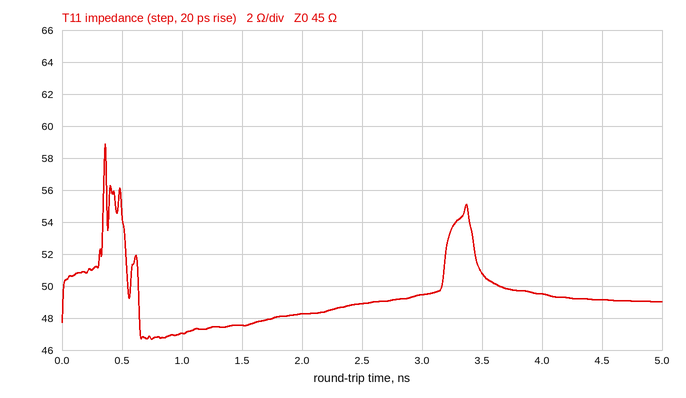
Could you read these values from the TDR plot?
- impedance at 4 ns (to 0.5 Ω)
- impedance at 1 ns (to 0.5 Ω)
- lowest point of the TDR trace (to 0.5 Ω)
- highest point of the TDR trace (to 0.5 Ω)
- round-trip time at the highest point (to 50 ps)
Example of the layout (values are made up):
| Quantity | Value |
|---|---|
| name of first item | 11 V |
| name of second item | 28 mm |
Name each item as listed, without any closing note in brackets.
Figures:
| Quantity | Value |
|---|---|
| impedance at 4 ns | 49.5 Ω |
| impedance at 1 ns | 47.0 Ω |
| lowest point of the TDR trace | 46.5 Ω |
| highest point of the TDR trace | 59.0 Ω |
| round-trip time at the highest point | 350 ps |
